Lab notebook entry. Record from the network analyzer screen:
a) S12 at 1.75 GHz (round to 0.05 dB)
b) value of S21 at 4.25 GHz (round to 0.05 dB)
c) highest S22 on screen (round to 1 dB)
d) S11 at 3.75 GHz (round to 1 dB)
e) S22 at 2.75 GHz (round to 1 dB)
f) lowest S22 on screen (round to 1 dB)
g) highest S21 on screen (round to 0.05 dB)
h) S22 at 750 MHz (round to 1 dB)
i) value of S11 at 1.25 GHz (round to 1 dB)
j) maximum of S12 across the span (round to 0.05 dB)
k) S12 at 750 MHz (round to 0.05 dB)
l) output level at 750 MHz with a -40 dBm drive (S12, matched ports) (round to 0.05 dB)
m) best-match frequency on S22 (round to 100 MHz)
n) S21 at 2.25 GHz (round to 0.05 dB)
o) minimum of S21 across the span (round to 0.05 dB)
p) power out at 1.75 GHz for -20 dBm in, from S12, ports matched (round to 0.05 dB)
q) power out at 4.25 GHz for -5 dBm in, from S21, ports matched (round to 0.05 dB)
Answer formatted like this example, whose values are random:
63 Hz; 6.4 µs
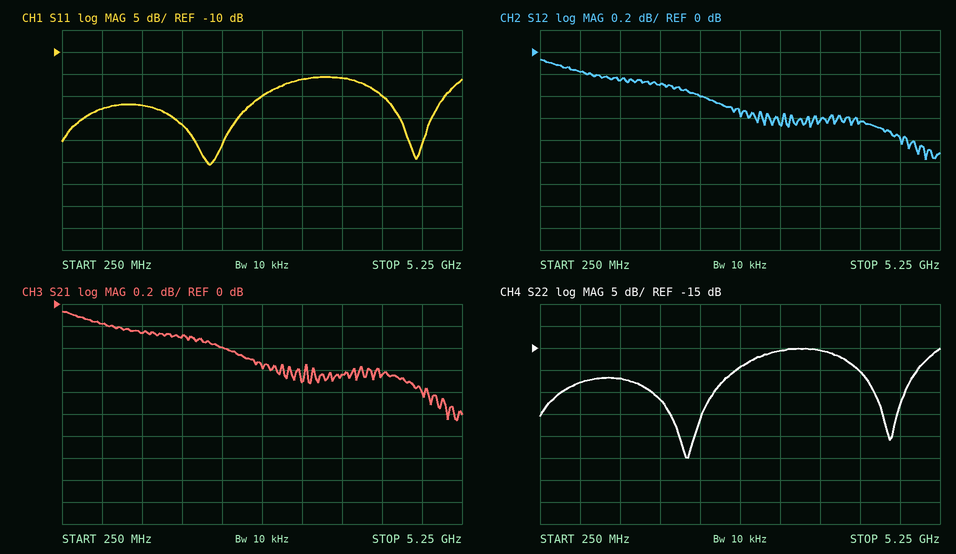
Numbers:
-0.30 dB; -0.65 dB; -15 dB; -16 dB; -19 dB; -40 dB; -0.05 dB; -23 dB; -22 dB; -0.05 dB; -0.20 dB; -40.20 dBm; 2.1 GHz; -0.40 dB; -1.05 dB; -20.30 dBm; -5.65 dBm
